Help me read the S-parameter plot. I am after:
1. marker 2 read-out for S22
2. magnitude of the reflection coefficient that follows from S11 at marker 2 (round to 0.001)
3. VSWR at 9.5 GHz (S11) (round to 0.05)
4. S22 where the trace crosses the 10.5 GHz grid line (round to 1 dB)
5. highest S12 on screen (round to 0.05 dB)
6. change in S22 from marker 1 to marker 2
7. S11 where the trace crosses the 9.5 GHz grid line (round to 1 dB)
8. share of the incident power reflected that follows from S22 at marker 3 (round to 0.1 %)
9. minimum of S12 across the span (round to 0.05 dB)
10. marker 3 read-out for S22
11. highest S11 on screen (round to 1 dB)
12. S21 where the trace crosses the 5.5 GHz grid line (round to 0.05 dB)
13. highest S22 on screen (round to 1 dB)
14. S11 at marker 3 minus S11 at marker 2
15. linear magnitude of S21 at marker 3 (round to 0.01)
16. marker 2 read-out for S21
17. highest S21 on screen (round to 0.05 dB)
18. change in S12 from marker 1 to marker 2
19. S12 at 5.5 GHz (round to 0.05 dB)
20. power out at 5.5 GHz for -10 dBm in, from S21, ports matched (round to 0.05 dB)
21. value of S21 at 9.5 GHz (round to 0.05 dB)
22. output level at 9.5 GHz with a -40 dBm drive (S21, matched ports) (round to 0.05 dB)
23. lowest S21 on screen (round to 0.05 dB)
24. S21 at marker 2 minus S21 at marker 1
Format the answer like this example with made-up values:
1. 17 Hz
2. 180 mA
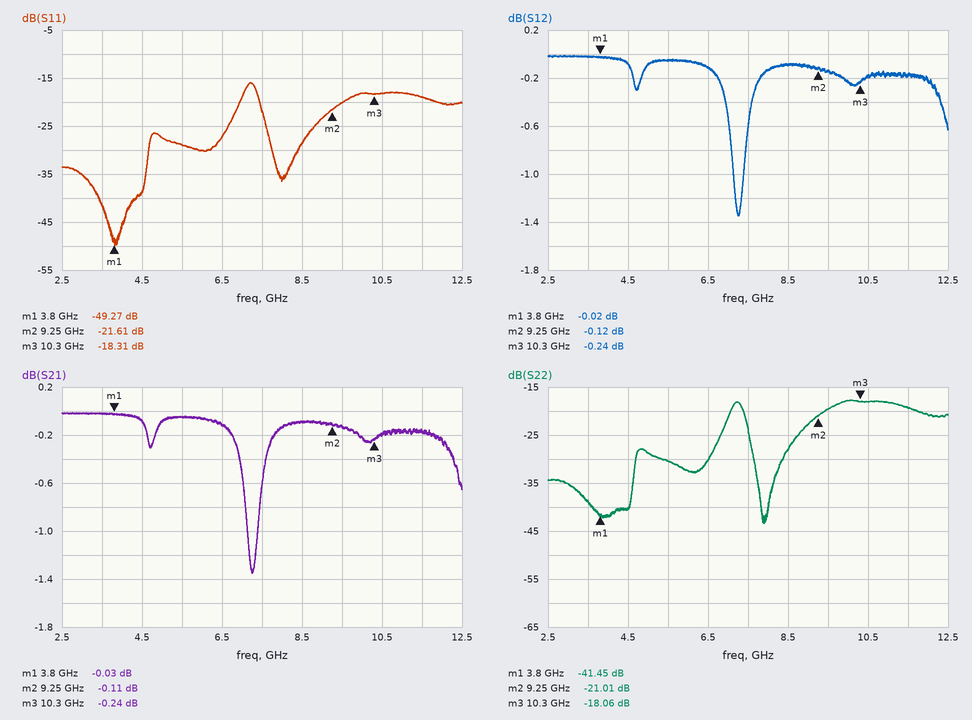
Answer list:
1. -21.01 dB
2. 0.083
3. 1.20
4. -18 dB
5. 0.00 dB
6. 20.44 dB
7. -20 dB
8. 1.6 %
9. -1.35 dB
10. -18.06 dB
11. -16 dB
12. -0.05 dB
13. -18 dB
14. 3.30 dB
15. 0.97
16. -0.11 dB
17. 0.00 dB
18. -0.10 dB
19. -0.05 dB
20. -10.05 dBm
21. -0.15 dB
22. -40.15 dBm
23. -1.35 dB
24. -0.08 dB
